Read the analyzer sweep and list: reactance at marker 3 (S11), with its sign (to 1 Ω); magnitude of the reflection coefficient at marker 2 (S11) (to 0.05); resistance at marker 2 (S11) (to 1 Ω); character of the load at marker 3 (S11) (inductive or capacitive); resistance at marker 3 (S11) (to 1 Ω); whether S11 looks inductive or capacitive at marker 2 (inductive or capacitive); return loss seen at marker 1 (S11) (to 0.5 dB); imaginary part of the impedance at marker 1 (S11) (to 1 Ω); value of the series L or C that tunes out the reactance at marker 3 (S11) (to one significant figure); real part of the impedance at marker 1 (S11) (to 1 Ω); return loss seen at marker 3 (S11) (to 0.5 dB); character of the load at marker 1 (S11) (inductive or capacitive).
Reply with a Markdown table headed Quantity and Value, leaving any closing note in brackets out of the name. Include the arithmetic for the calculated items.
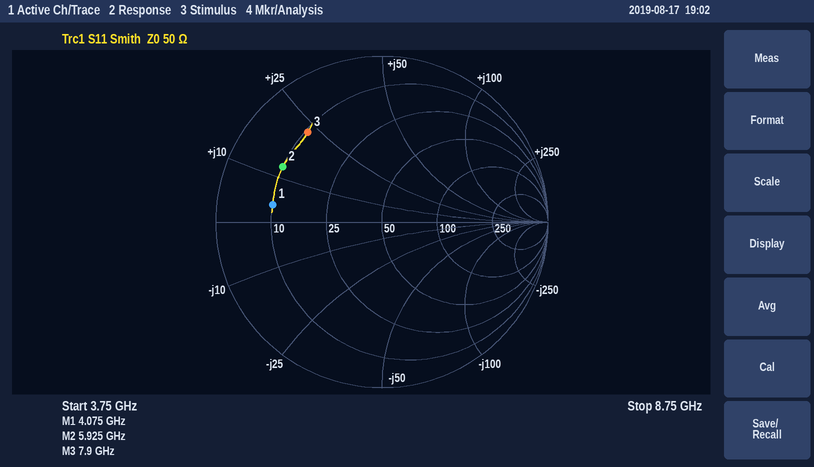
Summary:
| Quantity | Value |
|---|---|
| reactance at marker 3 (S11), with its sign | +23 Ω |
| magnitude of the reflection coefficient at marker 2 (S11) | 0.70 |
| resistance at marker 2 (S11) | 10 Ω |
| character of the load at marker 3 (S11) | inductive |
| resistance at marker 3 (S11) | 11 Ω |
| whether S11 looks inductive or capacitive at marker 2 | inductive |
| return loss seen at marker 1 (S11) | 3.5 dB |
| imaginary part of the impedance at marker 1 (S11) | +4 Ω |
| value of the series L or C that tunes out the reactance at marker 3 (S11) | C = 1/(2π × 7.9 GHz × 23 Ω) ≈ 876 fF, so 900 fF to one significant figure |
| real part of the impedance at marker 1 (S11) | 10 Ω |
| return loss seen at marker 3 (S11) | 3.0 dB |
| character of the load at marker 1 (S11) | inductive |
